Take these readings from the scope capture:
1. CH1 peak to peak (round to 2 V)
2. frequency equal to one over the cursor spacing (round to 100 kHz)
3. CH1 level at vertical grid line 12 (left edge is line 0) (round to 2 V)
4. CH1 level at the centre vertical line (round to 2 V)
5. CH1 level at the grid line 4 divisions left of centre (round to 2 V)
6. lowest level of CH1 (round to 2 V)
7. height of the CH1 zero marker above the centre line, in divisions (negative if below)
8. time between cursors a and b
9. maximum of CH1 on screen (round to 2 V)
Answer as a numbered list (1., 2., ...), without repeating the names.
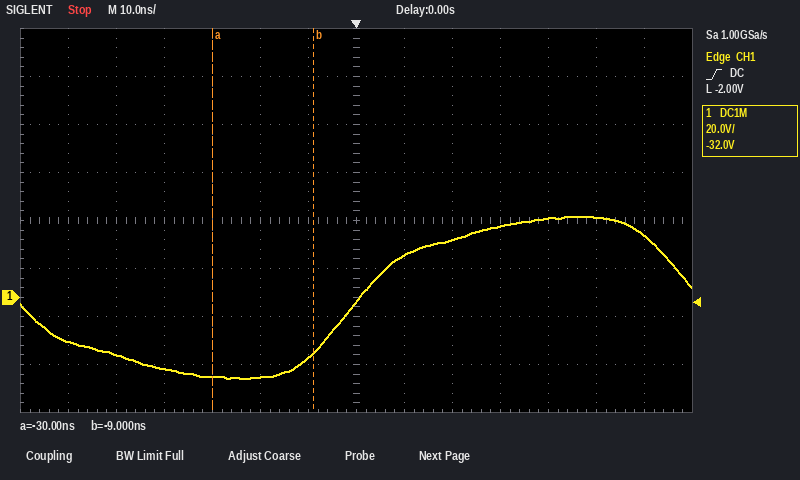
1. 68 V
2. 47.6 MHz
3. 34 V
4. -2 V
5. -30 V
6. -34 V
7. -1.6 div
8. 21 ns
9. 34 V
